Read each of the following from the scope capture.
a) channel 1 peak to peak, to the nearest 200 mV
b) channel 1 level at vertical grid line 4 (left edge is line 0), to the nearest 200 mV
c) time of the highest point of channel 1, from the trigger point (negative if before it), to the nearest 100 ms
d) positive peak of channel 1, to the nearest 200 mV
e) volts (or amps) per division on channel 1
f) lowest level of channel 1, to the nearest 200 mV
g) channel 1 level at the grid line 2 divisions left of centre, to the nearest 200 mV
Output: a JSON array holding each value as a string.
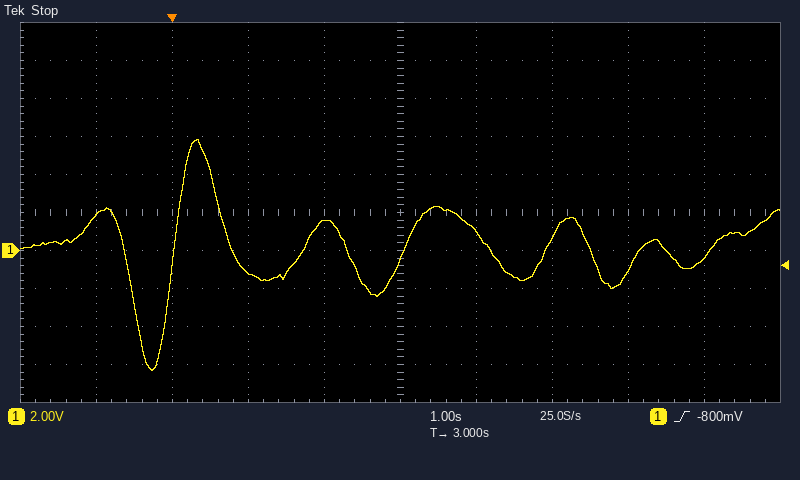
["12.2 V", "1.6 V", "+300 ms", "5.8 V", "2 V", "-6.4 V", "-1.2 V"]
